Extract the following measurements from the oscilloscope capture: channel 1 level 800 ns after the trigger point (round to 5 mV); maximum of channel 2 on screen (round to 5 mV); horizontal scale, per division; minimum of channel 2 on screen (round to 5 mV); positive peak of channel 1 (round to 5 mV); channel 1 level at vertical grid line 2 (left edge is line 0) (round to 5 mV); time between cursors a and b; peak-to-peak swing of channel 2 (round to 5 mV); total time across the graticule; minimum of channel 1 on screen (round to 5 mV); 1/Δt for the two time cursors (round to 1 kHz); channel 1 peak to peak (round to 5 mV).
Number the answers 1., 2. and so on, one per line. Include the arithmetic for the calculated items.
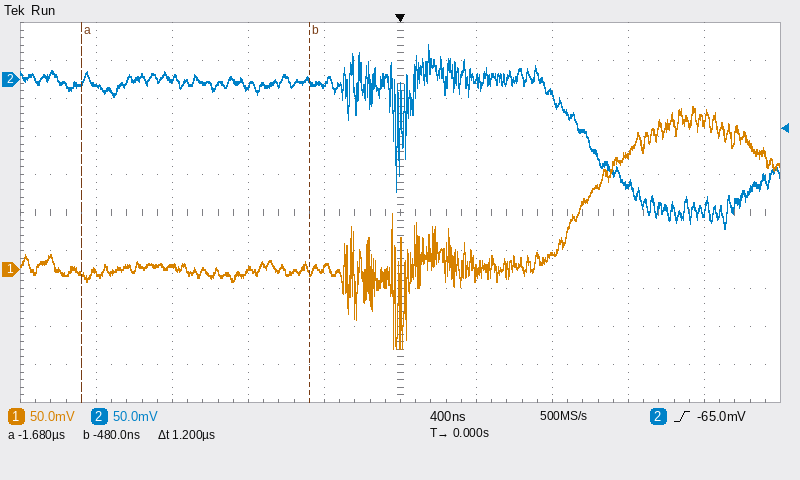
1. 20 mV
2. 45 mV
3. 400 ns
4. -195 mV
5. 215 mV
6. 5 mV
7. 1.2 µs
8. 45 mV − (-195 mV) = 240 mV
9. 4 µs
10. -105 mV
11. 1 / 1.2 µs ≈ 833 kHz
12. 215 mV − (-105 mV) = 320 mV
